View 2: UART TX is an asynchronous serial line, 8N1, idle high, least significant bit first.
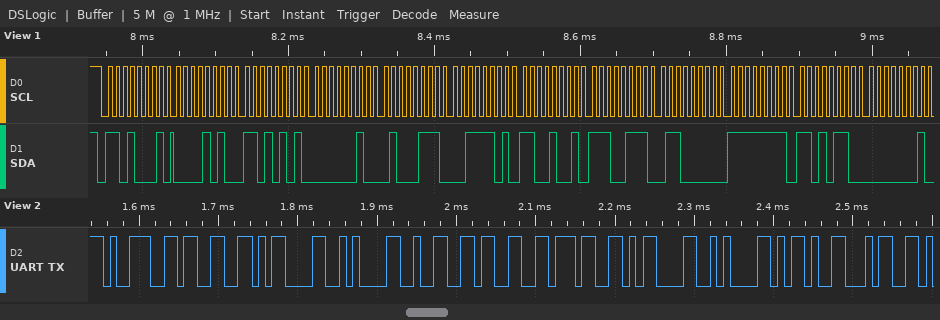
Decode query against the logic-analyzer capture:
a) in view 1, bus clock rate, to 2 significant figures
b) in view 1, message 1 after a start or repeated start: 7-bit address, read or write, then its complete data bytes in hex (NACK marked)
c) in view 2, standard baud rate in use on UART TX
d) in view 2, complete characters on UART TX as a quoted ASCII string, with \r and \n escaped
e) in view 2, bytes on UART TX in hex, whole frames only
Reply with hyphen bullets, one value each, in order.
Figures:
- 100 kHz
- 0x68 read: 0A D5 02 47 3D C9 E7 60 FF D6 01
- 115200 baud
- "93\r\n237\r\n-4"
- 39 33 0D 0A 32 33 37 0D 0A 2D 34
